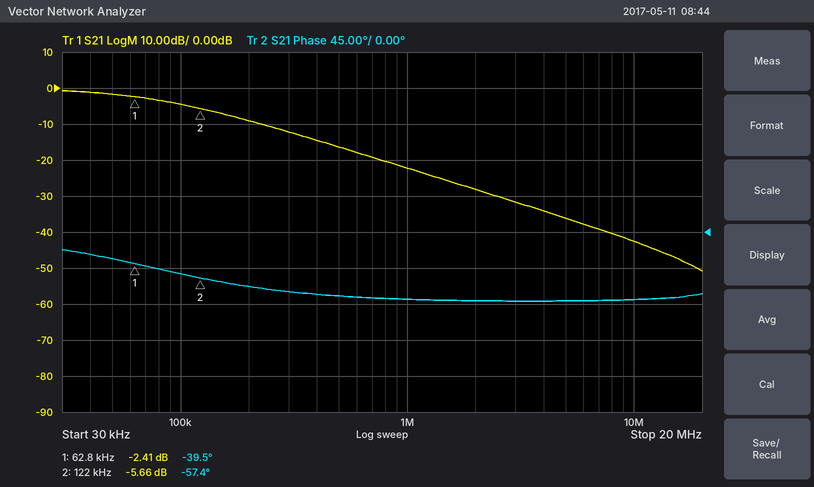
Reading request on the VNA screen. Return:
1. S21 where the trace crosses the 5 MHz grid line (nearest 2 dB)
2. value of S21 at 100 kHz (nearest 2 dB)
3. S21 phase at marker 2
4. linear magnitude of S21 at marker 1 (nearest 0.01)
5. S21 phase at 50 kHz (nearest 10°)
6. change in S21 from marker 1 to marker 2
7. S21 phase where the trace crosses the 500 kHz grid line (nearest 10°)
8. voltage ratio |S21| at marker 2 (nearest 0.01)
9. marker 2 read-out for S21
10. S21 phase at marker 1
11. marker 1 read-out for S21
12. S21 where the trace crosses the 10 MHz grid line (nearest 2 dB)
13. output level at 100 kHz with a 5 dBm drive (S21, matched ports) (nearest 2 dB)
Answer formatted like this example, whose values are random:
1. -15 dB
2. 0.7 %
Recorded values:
1. -36 dB
2. -4 dB
3. -57.4°
4. 0.76
5. -30°
6. -3.25 dB
7. -80°
8. 0.52
9. -5.66 dB
10. -39.5°
11. -2.41 dB
12. -42 dB
13. 0 dBm
